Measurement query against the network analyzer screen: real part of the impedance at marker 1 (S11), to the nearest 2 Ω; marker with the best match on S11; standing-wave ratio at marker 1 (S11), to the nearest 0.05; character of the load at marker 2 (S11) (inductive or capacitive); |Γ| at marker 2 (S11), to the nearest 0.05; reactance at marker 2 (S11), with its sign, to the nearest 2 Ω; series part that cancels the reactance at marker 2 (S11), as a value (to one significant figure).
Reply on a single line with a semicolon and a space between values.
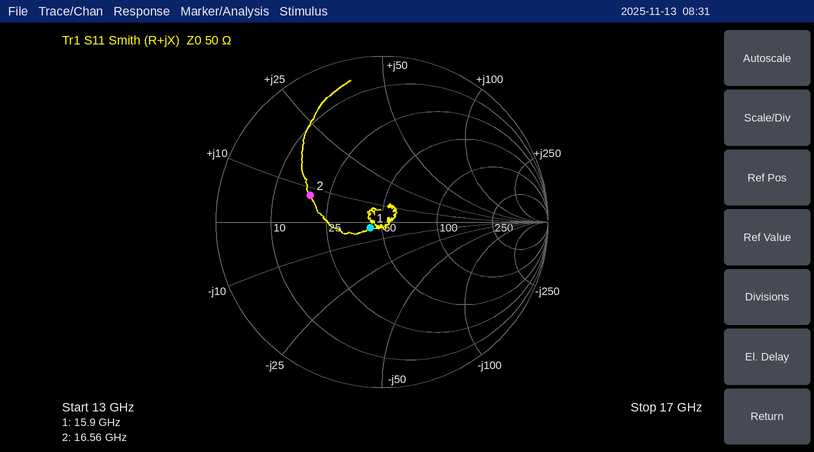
44 Ω; marker 1; 1.15; inductive; 0.45; +8 Ω; 1 pF
